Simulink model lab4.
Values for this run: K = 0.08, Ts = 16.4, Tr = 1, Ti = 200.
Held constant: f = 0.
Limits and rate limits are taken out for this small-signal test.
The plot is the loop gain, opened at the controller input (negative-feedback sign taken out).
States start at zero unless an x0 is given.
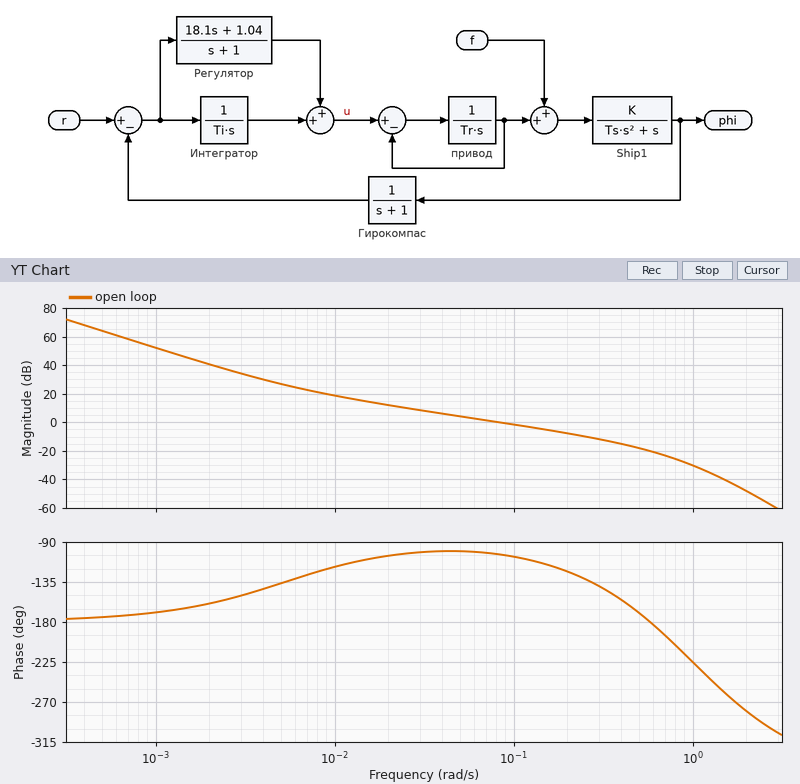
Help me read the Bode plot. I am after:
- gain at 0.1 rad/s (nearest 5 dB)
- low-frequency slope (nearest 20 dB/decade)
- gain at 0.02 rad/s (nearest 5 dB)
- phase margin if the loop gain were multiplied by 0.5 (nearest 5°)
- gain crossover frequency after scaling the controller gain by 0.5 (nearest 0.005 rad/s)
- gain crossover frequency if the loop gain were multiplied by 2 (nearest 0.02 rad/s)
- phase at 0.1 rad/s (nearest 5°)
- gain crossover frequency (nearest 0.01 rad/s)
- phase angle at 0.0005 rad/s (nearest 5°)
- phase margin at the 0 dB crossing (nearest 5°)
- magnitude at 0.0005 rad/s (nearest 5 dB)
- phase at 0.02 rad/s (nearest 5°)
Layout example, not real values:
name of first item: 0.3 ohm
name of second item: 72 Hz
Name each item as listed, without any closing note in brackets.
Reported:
gain at 0.1 rad/s: 0 dB
low-frequency slope: -40 dB/decade
gain at 0.02 rad/s: 10 dB
phase margin if the loop gain were multiplied by 0.5: 80°
gain crossover frequency after scaling the controller gain by 0.5: 0.040 rad/s
gain crossover frequency if the loop gain were multiplied by 2: 0.16 rad/s
phase at 0.1 rad/s: -105°
gain crossover frequency: 0.08 rad/s
phase angle at 0.0005 rad/s: -175°
phase margin at the 0 dB crossing: 75°
magnitude at 0.0005 rad/s: 65 dB
phase at 0.02 rad/s: -105°
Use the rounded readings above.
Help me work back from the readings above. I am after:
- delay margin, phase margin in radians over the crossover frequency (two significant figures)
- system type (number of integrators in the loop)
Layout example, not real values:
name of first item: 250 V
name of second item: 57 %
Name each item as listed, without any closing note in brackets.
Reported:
delay margin, phase margin in radians over the crossover frequency: 16 s
system type: 2
